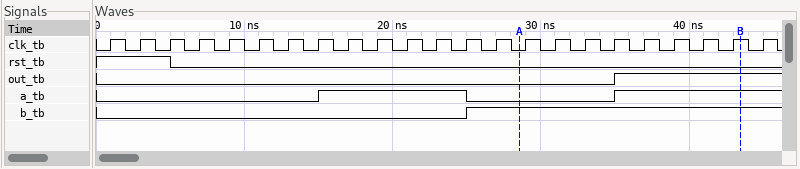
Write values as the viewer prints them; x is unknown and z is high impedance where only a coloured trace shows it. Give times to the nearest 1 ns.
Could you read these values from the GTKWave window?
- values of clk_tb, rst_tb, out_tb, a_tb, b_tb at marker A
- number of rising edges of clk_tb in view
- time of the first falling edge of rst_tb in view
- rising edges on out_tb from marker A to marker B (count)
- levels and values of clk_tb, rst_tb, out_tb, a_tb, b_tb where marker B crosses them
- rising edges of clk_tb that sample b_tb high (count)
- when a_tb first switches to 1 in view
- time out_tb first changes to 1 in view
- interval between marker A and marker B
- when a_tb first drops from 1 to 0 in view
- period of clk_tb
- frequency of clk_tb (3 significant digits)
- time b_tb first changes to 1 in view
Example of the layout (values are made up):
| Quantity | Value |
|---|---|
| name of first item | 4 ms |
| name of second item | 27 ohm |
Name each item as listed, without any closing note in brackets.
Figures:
| Quantity | Value |
|---|---|
| values of clk_tb, rst_tb, out_tb, a_tb, b_tb at marker A | clk_tb=0, rst_tb=0, out_tb=0, a_tb=0, b_tb=1 |
| number of rising edges of clk_tb in view | 23 |
| time of the first falling edge of rst_tb in view | 5 ns |
| rising edges on out_tb from marker A to marker B | 1 |
| levels and values of clk_tb, rst_tb, out_tb, a_tb, b_tb where marker B crosses them | clk_tb=1, rst_tb=0, out_tb=1, a_tb=1, b_tb=1 |
| rising edges of clk_tb that sample b_tb high | 10 |
| when a_tb first switches to 1 in view | 15 ns |
| time out_tb first changes to 1 in view | 35 ns |
| interval between marker A and marker B | 15 ns |
| when a_tb first drops from 1 to 0 in view | 25 ns |
| period of clk_tb | 2 ns |
| frequency of clk_tb | 500 MHz |
| time b_tb first changes to 1 in view | 25 ns |
